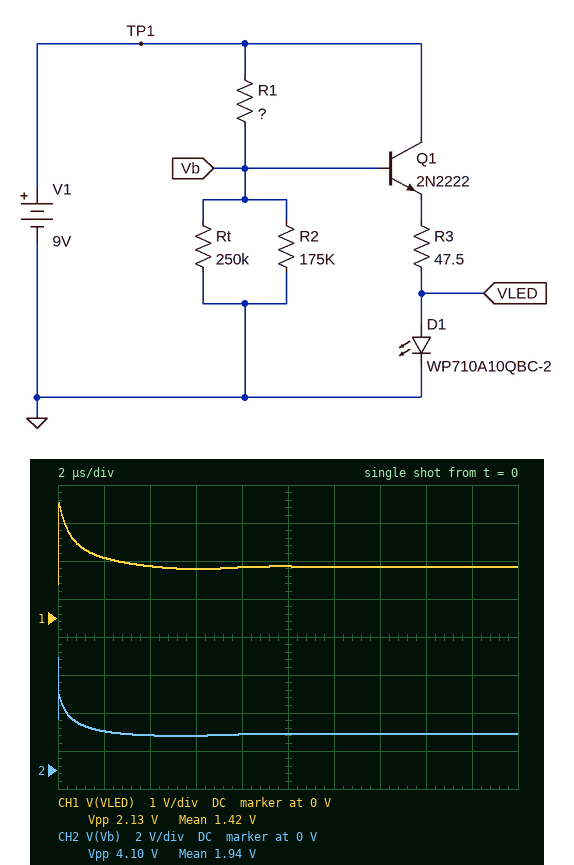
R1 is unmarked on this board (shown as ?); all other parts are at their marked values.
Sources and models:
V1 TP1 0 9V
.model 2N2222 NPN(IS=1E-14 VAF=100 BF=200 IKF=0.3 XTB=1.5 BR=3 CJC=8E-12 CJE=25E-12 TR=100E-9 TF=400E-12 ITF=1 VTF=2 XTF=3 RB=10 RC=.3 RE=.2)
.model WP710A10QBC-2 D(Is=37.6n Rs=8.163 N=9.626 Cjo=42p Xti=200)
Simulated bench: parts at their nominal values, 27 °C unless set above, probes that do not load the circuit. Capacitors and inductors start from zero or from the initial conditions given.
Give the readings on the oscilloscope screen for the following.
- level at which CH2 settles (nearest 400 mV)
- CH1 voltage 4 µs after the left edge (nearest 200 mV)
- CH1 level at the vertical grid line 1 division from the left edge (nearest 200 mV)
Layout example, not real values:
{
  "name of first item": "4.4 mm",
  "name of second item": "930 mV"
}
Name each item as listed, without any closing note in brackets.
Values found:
{
  "level at which CH2 settles": "2.0 V",
  "CH1 voltage 4 µs after the left edge": "1.4 V",
  "CH1 level at the vertical grid line 1 division from the left edge": "1.6 V"
}
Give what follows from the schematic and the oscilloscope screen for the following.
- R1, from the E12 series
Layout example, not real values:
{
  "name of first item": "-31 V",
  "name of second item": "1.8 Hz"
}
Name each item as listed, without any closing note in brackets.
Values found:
{
  "R1, from the E12 series": "390 kΩ"
}
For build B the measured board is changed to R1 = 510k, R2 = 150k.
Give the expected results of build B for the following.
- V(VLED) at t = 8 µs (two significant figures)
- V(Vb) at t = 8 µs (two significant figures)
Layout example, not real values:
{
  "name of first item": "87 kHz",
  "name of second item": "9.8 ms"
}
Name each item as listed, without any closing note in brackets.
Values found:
{
  "V(VLED) at t = 8 µs": "1.1 V",
  "V(Vb) at t = 8 µs": "1.3 V"
}
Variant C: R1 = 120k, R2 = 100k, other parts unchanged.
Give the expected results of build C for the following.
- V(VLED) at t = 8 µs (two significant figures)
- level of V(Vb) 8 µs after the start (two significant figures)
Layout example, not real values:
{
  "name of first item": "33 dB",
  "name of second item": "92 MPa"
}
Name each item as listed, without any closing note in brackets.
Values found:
{
  "V(VLED) at t = 8 µs": "2.5 V",
  "level of V(Vb) 8 µs after the start": "3.2 V"
}
